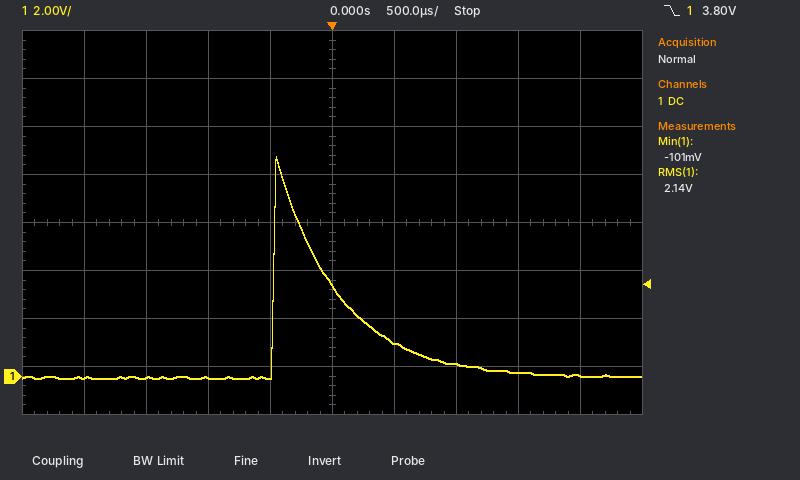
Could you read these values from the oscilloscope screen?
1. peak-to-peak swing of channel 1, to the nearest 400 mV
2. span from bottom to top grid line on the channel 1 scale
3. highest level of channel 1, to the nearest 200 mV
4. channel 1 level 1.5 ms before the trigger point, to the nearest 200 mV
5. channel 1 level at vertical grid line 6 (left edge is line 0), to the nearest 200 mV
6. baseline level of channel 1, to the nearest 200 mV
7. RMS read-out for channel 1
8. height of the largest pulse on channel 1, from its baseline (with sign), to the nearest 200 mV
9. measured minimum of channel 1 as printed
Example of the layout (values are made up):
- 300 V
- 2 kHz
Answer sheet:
- 9.2 V
- 16 V
- 9.2 V
- 0.0 V
- 1.4 V
- 0.0 V
- 2.14 V
- +9.2 V
- -101 mV
